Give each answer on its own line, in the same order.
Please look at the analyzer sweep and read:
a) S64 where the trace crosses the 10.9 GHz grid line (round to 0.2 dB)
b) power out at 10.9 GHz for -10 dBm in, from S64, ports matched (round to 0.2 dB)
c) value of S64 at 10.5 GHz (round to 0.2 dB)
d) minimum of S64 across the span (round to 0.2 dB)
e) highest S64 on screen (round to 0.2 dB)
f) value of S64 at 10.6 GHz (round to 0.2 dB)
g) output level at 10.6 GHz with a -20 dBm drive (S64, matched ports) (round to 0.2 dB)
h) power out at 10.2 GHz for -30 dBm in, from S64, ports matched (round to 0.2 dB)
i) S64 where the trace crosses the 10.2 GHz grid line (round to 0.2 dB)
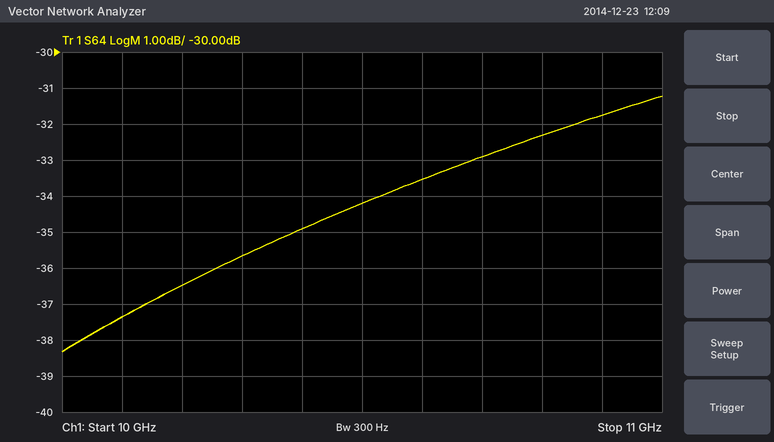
-31.8 dB
-41.8 dBm
-34.2 dB
-38.4 dB
-31.2 dB
-33.6 dB
-53.6 dBm
-66.4 dBm
-36.4 dB
